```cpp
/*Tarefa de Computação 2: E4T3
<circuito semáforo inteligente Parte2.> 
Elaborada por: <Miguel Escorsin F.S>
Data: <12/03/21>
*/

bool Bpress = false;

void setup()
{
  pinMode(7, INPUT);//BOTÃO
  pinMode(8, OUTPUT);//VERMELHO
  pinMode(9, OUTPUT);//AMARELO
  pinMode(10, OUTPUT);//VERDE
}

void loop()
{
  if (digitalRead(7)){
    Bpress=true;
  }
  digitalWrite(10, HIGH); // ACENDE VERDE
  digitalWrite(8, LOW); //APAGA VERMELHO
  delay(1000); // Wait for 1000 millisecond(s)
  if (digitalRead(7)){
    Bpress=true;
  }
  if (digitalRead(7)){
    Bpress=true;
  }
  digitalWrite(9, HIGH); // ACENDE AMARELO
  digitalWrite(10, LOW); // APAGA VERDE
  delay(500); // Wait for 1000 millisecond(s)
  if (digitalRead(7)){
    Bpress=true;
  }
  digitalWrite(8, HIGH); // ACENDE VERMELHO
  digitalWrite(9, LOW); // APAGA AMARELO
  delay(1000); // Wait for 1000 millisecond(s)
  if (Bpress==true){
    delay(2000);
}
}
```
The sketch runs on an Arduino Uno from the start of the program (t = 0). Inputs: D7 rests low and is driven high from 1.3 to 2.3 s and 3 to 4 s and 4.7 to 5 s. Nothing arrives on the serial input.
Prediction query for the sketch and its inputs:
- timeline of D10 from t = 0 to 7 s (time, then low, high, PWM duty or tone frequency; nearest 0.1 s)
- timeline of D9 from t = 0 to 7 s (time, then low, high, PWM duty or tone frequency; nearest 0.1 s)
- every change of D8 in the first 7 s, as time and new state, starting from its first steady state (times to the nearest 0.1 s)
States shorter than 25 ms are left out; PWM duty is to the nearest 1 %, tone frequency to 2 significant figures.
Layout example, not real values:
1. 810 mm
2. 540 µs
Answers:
1. 0 s high; 1 s low; 4.5 s high; 5.5 s low
2. 0 s low; 1 s high; 1.5 s low; 5.5 s high; 6 s low
3. 0 s low; 1.5 s high; 4.5 s low; 6 s high
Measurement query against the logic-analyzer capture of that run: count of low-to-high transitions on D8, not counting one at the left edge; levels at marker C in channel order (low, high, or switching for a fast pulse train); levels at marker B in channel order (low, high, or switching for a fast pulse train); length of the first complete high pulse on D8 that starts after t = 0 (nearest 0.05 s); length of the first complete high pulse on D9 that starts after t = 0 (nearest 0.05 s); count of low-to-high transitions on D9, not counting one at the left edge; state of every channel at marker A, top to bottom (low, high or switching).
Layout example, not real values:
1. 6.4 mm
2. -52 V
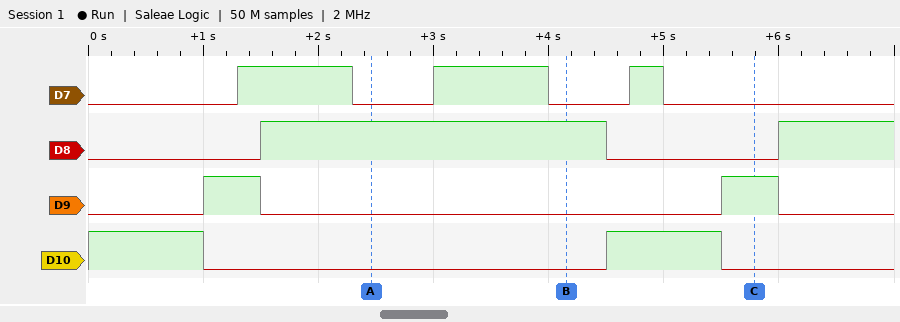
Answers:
1. 2
2. D7 low, D8 low, D9 high, D10 low
3. D7 low, D8 high, D9 low, D10 low
4. 3.00 s
5. 0.50 s
6. 2
7. D7 low, D8 high, D9 low, D10 low
